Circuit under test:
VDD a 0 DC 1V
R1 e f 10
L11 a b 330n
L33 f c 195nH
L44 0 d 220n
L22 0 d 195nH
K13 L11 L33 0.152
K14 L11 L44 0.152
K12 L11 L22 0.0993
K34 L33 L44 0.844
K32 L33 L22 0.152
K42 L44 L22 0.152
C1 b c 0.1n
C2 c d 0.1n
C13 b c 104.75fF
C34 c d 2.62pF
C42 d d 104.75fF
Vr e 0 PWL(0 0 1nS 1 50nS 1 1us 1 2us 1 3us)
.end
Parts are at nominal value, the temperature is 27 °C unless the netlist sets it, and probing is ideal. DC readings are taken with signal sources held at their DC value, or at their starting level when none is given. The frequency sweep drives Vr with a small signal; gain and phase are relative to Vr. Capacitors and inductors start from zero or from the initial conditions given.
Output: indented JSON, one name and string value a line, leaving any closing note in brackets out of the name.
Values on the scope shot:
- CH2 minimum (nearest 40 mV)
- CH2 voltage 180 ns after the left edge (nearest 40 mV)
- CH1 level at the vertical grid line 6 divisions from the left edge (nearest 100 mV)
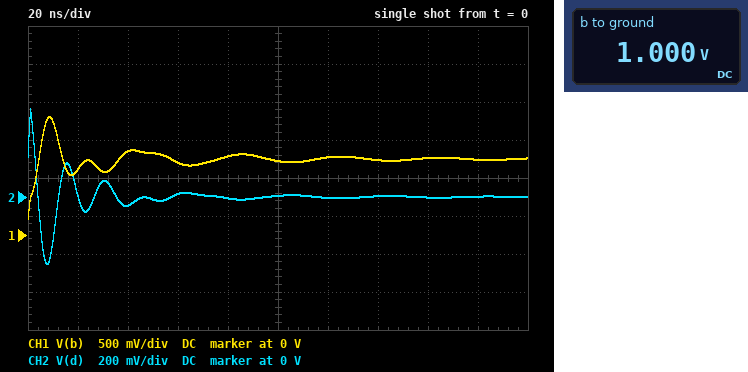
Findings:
{
  "CH2 minimum": "-360 mV",
  "CH2 voltage 180 ns after the left edge": "0 V",
  "CH1 level at the vertical grid line 6 divisions from the left edge": "1.0 V"
}
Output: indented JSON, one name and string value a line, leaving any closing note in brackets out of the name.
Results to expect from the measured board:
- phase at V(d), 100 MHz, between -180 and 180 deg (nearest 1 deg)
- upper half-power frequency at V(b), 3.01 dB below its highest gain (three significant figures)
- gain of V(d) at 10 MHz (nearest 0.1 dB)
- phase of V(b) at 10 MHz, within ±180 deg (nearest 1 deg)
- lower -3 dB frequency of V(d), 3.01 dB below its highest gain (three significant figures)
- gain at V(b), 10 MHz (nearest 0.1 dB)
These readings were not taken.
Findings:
{
  "phase at V(d), 100 MHz, between -180 and 180 deg": "24 deg",
  "upper half-power frequency at V(b), 3.01 dB below its highest gain": "28.7 MHz",
  "gain of V(d) at 10 MHz": "-33.4 dB",
  "phase of V(b) at 10 MHz, within ±180 deg": "172 deg",
  "lower -3 dB frequency of V(d), 3.01 dB below its highest gain": "55.4 MHz",
  "gain at V(b), 10 MHz": "-17.0 dB"
}
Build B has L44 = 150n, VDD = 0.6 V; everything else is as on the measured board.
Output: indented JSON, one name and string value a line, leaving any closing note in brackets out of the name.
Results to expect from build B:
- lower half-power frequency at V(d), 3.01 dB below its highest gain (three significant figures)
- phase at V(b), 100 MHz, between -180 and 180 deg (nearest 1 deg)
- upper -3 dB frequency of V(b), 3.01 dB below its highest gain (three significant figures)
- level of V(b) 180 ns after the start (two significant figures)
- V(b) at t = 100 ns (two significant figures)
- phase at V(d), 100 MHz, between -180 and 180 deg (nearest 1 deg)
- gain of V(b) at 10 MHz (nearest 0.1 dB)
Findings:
{
  "lower half-power frequency at V(d), 3.01 dB below its highest gain": "23.1 MHz",
  "phase at V(b), 100 MHz, between -180 and 180 deg": "-152 deg",
  "upper -3 dB frequency of V(b), 3.01 dB below its highest gain": "28.5 MHz",
  "level of V(b) 180 ns after the start": "580 mV",
  "V(b) at t = 100 ns": "520 mV",
  "phase at V(d), 100 MHz, between -180 and 180 deg": "28 deg",
  "gain of V(b) at 10 MHz": "-17.2 dB"
}
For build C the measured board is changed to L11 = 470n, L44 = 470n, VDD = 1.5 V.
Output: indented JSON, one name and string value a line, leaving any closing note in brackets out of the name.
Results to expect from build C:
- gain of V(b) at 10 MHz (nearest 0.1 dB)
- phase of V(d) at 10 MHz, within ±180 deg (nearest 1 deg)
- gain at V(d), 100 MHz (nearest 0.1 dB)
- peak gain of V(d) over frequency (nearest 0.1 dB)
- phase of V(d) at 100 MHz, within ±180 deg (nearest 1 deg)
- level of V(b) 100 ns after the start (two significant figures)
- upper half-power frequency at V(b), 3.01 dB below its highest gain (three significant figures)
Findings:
{
  "gain of V(b) at 10 MHz": "-13.1 dB",
  "phase of V(d) at 10 MHz, within ±180 deg": "172 deg",
  "gain at V(d), 100 MHz": "-0.1 dB",
  "peak gain of V(d) over frequency": "8.3 dB",
  "phase of V(d) at 100 MHz, within ±180 deg": "15 deg",
  "level of V(b) 100 ns after the start": "1.6 V",
  "upper half-power frequency at V(b), 3.01 dB below its highest gain": "24.6 MHz"
}
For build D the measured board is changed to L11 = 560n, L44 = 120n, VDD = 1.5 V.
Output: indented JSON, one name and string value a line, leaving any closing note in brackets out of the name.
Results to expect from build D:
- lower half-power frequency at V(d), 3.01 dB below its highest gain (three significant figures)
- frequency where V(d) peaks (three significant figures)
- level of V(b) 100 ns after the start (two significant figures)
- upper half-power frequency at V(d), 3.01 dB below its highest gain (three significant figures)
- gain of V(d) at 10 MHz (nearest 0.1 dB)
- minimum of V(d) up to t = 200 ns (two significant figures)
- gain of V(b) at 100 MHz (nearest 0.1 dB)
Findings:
{
  "lower half-power frequency at V(d), 3.01 dB below its highest gain": "19.0 MHz",
  "frequency where V(d) peaks": "20.4 MHz",
  "level of V(b) 100 ns after the start": "1.4 V",
  "upper half-power frequency at V(d), 3.01 dB below its highest gain": "22.1 MHz",
  "gain of V(d) at 10 MHz": "-29.6 dB",
  "minimum of V(d) up to t = 200 ns": "-53 mV",
  "gain of V(b) at 100 MHz": "-0.5 dB"
}
